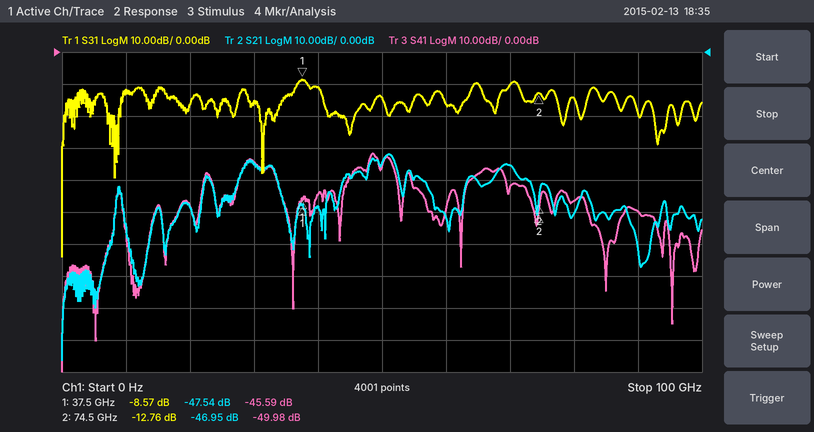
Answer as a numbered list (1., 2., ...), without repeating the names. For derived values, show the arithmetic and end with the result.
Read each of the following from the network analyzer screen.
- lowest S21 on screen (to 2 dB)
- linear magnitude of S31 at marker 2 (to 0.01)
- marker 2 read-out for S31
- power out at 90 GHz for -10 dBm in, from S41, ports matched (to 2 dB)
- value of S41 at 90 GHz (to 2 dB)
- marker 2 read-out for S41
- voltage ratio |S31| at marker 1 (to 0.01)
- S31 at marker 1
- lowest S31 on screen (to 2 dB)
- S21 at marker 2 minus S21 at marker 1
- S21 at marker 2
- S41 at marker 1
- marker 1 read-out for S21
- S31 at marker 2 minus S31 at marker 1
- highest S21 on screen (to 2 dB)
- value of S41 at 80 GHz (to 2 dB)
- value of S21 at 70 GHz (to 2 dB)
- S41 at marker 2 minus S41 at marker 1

1. -96 dB
2. 10^(-12.76/20) ≈ 0.23
3. -12.76 dB
4. -10 dBm + (-50 dB) = -60 dBm
5. -50 dB
6. -49.98 dB
7. 10^(-8.57/20) ≈ 0.37
8. -8.57 dB
9. -64 dB
10. -46.95 − (-47.54) = 0.59 dB
11. -46.95 dB
12. -45.59 dB
13. -47.54 dB
14. -12.76 − (-8.57) = -4.19 dB
15. -32 dB
16. -46 dB
17. -36 dB
18. -49.98 − (-45.59) = -4.39 dB
